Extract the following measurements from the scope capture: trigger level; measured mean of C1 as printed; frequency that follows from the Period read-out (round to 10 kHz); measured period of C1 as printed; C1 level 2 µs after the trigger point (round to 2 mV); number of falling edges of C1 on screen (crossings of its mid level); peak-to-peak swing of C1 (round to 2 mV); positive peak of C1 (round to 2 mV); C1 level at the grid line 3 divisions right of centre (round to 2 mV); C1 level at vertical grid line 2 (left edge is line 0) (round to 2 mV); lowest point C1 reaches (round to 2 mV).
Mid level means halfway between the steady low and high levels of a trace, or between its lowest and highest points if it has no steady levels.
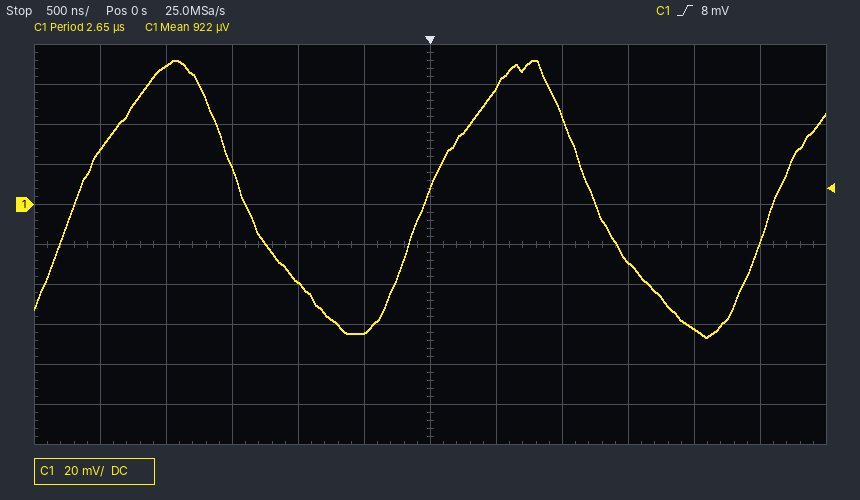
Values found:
8 mV
922 µV
380 kHz
2.65 µs
-62 mV
2
138 mV
72 mV
-28 mV
70 mV
-66 mV
